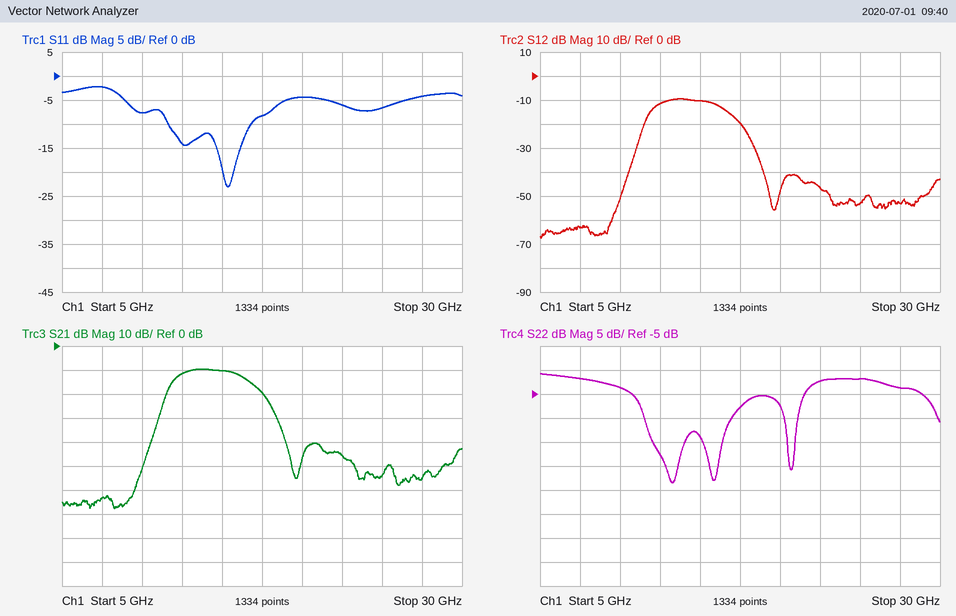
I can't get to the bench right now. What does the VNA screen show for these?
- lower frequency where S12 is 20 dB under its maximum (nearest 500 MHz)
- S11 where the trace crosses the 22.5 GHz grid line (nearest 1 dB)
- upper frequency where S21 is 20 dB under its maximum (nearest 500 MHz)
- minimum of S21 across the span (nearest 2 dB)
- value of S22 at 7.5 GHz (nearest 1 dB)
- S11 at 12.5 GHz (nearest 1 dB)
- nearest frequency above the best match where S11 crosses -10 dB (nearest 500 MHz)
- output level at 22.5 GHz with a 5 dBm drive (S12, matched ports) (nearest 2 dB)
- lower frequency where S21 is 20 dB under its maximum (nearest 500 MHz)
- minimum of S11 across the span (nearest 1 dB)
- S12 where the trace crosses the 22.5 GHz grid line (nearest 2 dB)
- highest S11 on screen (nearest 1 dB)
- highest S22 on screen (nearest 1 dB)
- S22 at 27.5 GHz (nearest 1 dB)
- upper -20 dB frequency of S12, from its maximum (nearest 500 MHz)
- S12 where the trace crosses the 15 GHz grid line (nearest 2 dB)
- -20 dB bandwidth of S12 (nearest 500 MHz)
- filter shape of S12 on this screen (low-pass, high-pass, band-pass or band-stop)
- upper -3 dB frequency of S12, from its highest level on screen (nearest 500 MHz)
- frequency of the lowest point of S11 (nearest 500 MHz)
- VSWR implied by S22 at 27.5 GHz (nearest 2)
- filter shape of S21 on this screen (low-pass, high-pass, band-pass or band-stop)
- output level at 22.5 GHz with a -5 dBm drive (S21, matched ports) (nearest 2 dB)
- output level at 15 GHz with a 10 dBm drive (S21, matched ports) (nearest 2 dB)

11.0 GHz
-6 dB
18.5 GHz
-68 dB
-2 dB
-14 dB
17.0 GHz
-42 dBm
11.0 GHz
-23 dB
-46 dB
-2 dB
-1 dB
-4 dB
18.5 GHz
-10 dB
7.5 GHz
band-pass
16.0 GHz
15.5 GHz
4
band-pass
-50 dBm
0 dBm
